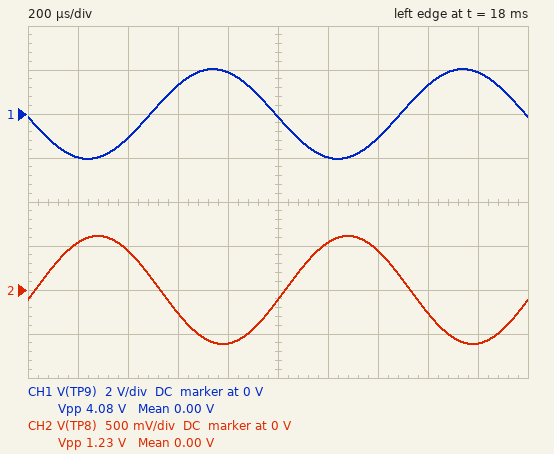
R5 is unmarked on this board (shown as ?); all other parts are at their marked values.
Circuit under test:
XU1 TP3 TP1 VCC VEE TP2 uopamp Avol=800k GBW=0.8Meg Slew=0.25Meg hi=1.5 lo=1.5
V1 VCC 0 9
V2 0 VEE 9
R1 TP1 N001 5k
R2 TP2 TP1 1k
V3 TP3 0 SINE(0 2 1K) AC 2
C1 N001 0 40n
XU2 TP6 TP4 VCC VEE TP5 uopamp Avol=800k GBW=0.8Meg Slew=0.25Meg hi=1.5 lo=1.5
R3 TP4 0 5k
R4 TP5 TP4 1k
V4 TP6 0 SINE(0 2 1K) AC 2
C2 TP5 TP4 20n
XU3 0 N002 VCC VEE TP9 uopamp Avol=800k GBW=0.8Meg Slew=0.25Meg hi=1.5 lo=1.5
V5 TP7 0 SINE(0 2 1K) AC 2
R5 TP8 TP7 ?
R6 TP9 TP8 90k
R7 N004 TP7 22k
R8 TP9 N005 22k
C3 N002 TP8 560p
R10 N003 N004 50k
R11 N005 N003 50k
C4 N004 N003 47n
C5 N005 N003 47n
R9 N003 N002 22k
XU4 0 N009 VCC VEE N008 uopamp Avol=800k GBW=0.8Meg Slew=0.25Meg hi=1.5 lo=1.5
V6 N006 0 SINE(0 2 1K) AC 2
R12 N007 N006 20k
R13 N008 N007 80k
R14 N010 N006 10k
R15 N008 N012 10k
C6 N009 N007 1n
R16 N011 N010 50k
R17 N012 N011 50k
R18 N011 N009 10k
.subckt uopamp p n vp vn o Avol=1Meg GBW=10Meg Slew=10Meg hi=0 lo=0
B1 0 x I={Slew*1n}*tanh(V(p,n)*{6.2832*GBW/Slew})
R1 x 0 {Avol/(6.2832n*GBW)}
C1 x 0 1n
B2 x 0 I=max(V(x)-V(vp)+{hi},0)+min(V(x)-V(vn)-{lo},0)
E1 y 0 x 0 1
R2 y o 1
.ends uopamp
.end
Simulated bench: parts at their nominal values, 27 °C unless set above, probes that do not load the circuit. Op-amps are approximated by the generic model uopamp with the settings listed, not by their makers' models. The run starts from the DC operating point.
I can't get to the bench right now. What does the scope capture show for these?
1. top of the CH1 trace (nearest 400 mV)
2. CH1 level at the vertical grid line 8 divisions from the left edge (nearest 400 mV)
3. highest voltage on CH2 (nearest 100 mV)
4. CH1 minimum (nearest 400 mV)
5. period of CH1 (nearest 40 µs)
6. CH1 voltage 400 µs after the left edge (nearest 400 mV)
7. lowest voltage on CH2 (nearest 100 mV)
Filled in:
2.0 V
1.2 V
600 mV
-2.0 V
1.00 ms
-1.2 V
-600 mV
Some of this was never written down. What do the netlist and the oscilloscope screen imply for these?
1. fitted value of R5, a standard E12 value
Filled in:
47 kΩ
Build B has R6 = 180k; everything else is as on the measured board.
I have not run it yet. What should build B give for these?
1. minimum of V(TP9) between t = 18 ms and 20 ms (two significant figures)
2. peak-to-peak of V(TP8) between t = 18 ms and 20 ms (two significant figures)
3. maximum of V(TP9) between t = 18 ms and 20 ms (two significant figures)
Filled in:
-2.1 V
2.3 V
2.1 V
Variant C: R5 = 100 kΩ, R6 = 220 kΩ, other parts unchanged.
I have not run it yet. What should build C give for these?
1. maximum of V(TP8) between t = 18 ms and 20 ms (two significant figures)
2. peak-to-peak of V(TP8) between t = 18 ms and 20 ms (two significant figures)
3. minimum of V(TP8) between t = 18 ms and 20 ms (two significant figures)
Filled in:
710 mV
1.4 V
-710 mV
